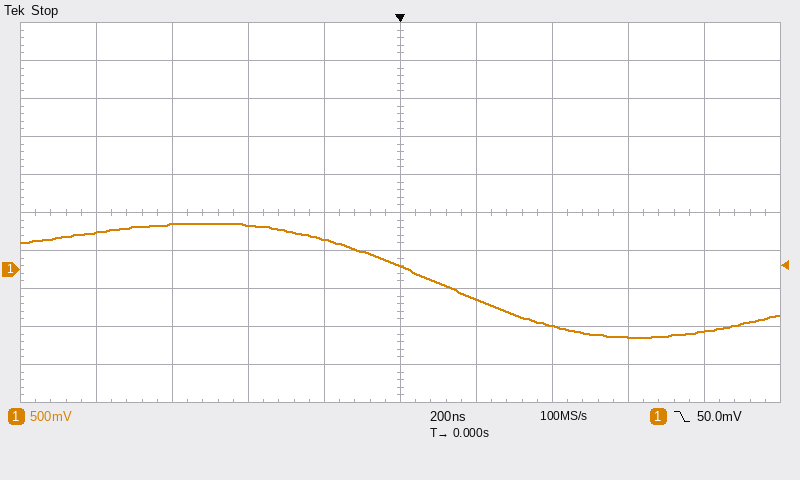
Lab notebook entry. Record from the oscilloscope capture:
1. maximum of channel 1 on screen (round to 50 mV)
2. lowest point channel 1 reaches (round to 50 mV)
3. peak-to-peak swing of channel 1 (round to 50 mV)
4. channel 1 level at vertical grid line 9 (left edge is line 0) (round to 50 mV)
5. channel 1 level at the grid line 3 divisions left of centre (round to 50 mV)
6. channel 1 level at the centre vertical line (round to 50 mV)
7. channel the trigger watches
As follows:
600 mV
-900 mV
1.50 V
-800 mV
600 mV
50 mV
channel 1
